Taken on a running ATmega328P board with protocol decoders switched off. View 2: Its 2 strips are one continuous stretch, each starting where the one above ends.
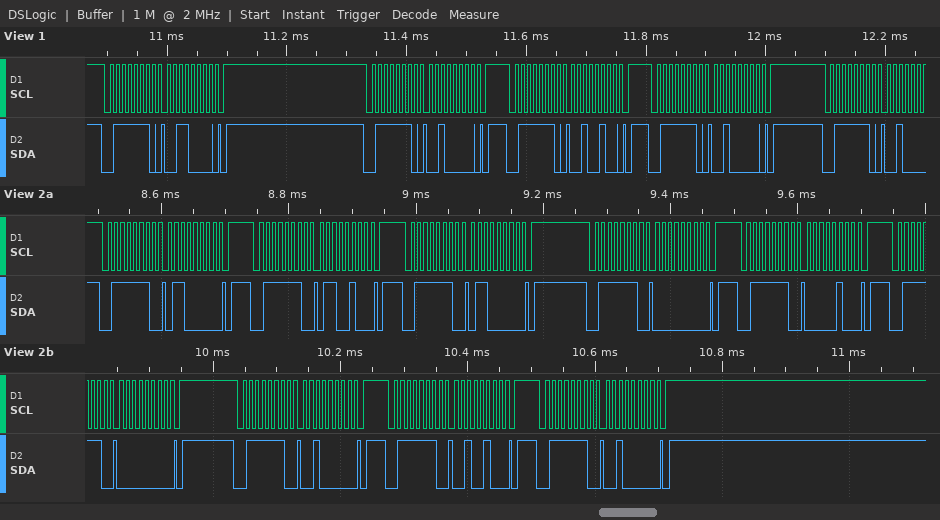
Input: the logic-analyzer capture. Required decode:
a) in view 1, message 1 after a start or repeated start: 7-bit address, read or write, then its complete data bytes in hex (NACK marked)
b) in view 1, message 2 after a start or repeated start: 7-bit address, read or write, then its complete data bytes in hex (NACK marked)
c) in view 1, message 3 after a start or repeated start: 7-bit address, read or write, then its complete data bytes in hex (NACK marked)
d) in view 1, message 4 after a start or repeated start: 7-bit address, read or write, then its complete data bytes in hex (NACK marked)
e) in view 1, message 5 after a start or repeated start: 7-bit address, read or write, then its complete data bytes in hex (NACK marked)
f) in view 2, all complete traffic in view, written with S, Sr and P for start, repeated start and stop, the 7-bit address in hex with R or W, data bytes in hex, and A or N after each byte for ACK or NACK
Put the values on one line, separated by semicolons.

0x3F write: 30; 0x3F write: 20; 0x3F write: 24; 0x3F write: 20; 0x3F write; S 3FW A 60 A P S 3FW A 64 A P S 3FW A 60 A P S 3FW A 00 A P S 3FW A 04 A P S 3FW A 00 A P S 3FW A 20 A P S 3FW A 24 A P S 3FW A 20 A P
